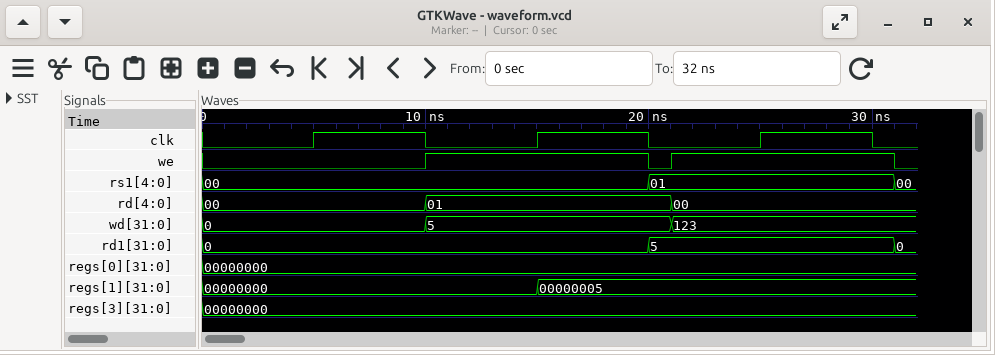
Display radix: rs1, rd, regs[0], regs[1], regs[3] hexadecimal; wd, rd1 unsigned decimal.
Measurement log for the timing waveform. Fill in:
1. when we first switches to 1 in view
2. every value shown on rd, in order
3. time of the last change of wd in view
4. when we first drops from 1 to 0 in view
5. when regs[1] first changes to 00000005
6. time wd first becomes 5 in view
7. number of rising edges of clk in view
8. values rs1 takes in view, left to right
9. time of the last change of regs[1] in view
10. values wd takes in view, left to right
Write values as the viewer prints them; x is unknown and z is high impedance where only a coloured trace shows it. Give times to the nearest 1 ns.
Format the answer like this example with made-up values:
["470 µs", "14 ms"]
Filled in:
["10 ns", "00, 01, 00", "21 ns", "20 ns", "15 ns", "10 ns", "3", "00, 01, 00", "15 ns", "0, 5, 123"]
